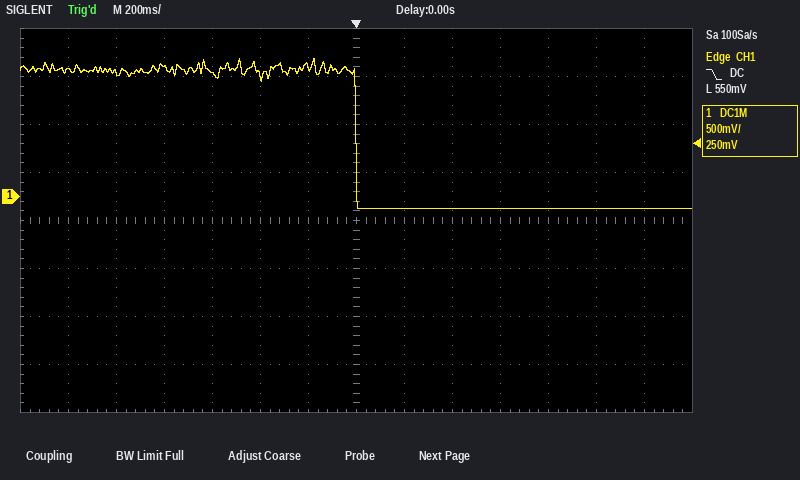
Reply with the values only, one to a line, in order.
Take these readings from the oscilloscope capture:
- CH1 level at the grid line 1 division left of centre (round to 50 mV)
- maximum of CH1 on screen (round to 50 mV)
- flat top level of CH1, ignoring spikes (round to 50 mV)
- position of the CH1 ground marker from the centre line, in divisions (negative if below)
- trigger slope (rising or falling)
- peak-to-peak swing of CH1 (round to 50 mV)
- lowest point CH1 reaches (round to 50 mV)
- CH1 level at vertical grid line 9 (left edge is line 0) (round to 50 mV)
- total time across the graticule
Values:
1.35 V
1.45 V
1.30 V
+0.5 div
falling
1.55 V
-100 mV
-100 mV
2.8 s
